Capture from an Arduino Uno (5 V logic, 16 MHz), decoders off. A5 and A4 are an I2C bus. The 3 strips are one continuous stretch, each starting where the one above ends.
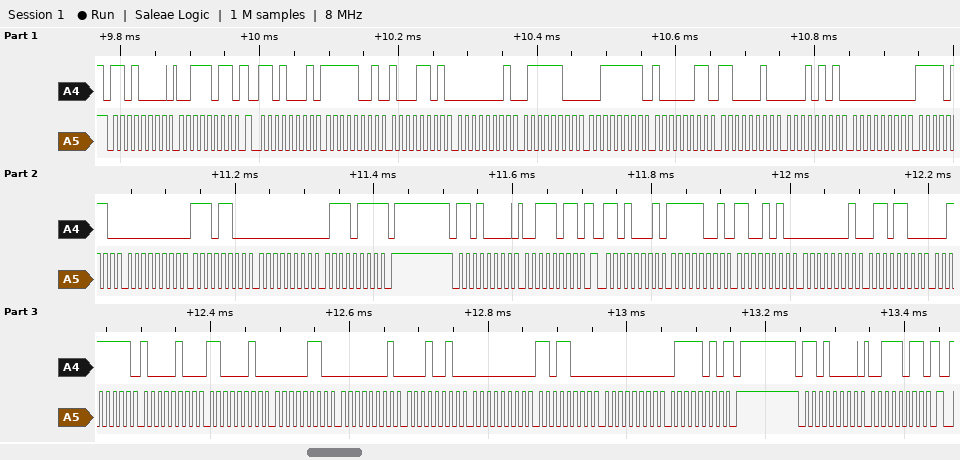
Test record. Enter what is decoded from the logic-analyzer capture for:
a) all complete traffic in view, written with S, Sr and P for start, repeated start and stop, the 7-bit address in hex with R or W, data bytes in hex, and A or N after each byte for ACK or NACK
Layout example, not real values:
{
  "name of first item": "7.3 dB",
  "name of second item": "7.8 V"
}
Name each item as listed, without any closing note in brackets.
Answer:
{
  "all complete traffic in view, written with S, Sr and P for start, repeated start and stop, the 7-bit address in hex with R or W, data bytes in hex, and A or N after each byte for ACK or NACK": "S 68W A 3B A Sr 68R A F9 A 8D A 01 A 7C A 3F A 83 A C2 A 15 A 00 A F6 A 00 A EC A 00 A 77 N P S 68W A 3B A Sr 68R A F9 A CA A 01 A 6C A 3F A 84 A C2 A 06 A 01 A 12 A 00 A D8 A 00 A 7A N P S 68W A 3B A"
}
